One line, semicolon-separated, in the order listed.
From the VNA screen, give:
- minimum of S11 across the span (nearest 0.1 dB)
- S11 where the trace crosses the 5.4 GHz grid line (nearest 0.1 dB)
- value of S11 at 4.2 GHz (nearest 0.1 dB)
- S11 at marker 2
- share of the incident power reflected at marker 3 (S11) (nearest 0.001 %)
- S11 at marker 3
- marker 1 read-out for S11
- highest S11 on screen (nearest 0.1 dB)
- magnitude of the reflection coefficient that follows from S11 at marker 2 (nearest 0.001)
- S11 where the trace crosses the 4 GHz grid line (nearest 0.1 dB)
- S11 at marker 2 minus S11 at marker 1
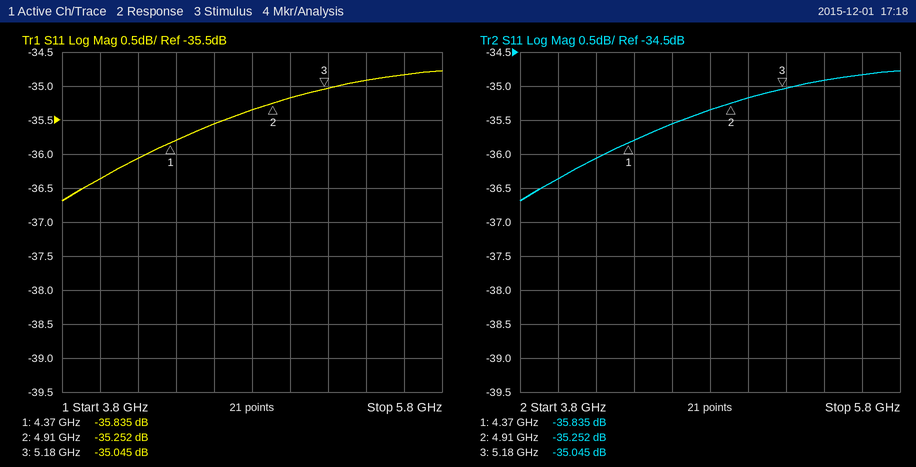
-36.7 dB; -34.9 dB; -36.1 dB; -35.252 dB; 0.031 %; -35.045 dB; -35.835 dB; -34.8 dB; 0.017; -36.4 dB; 0.583 dB
